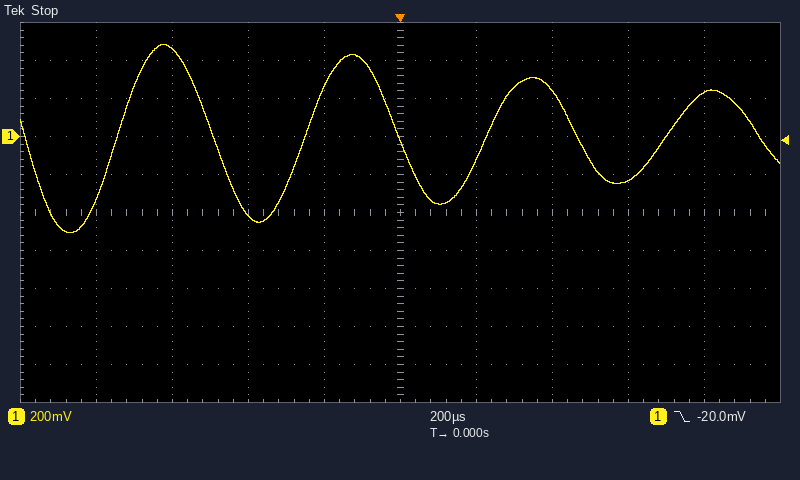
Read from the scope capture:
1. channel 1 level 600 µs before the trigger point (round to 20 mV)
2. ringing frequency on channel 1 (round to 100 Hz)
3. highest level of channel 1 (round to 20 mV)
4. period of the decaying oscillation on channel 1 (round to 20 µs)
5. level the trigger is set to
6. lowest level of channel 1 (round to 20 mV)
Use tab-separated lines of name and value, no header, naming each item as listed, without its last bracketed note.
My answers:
channel 1 level 600 µs before the trigger point	460 mV
ringing frequency on channel 1	2.1 kHz
highest level of channel 1	480 mV
period of the decaying oscillation on channel 1	480 µs
level the trigger is set to	-20.0 mV
lowest level of channel 1	-500 mV
